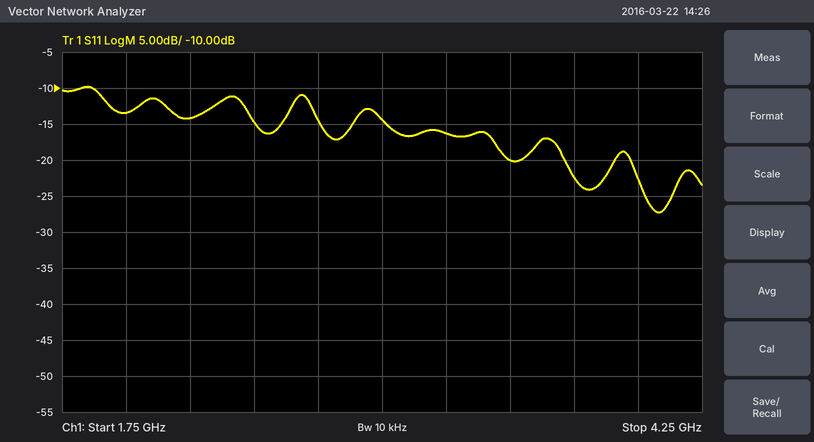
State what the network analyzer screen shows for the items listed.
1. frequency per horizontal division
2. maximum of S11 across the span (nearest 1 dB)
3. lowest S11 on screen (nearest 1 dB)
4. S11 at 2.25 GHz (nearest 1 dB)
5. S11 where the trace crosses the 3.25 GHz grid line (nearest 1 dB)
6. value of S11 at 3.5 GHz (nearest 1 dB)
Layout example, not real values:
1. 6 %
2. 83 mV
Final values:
1. 250 MHz
2. -10 dB
3. -27 dB
4. -14 dB
5. -16 dB
6. -20 dB
